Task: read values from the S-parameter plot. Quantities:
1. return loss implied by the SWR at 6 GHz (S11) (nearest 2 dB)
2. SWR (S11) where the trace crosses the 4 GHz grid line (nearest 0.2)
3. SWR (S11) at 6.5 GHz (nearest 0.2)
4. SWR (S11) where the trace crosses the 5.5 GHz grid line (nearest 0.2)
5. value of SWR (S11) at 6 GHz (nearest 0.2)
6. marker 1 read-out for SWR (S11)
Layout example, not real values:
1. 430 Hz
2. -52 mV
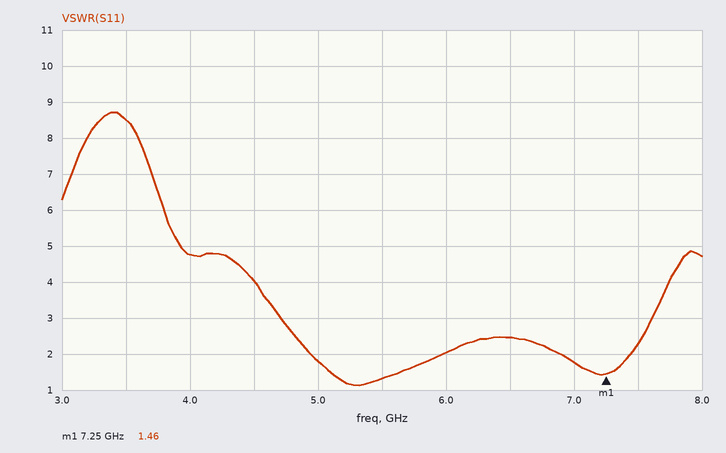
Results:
1. 10 dB
2. 4.8
3. 2.4
4. 1.4
5. 2.0
6. 1.46
